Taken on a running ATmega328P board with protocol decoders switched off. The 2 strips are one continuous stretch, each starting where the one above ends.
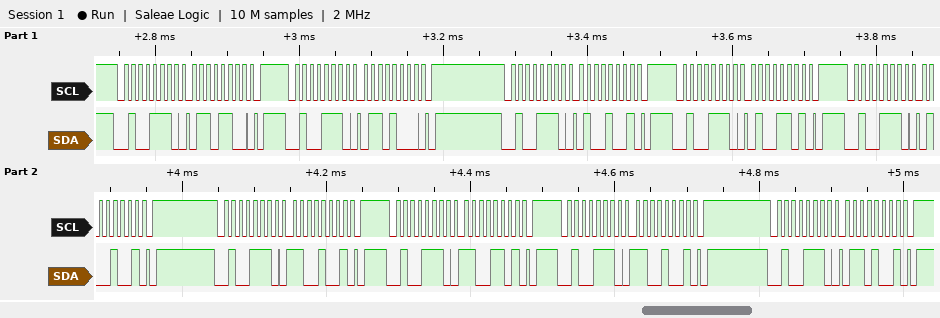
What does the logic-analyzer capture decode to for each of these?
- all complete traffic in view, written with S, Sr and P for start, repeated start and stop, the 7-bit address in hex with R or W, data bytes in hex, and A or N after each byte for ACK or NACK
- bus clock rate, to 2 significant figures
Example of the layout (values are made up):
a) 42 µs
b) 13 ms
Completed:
a) S 27W A 6C A P S 27W A 68 A P S 27W A 49 A P S 27W A 4D A P S 27W A 49 A P S 27W A C9 A P S 27W A CD A P S 27W A C9 A P S 27W A 69 A P
b) 100 kHz
